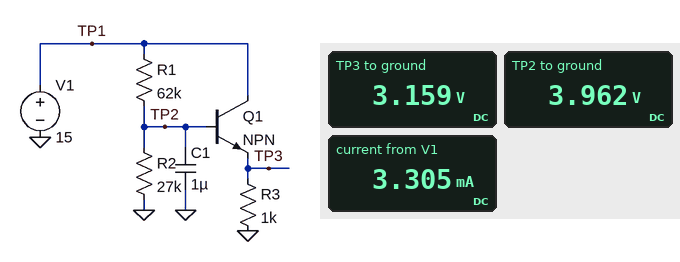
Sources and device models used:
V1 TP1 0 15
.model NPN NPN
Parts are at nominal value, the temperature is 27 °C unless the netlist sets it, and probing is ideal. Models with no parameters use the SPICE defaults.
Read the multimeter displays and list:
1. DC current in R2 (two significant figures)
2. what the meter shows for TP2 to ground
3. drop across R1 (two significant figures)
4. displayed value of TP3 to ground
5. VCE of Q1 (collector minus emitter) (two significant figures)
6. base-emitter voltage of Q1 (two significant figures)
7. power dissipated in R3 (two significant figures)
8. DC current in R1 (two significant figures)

150 µA
3.962 V
11 V
3.159 V
12 V
800 mV
10 mW
180 µA
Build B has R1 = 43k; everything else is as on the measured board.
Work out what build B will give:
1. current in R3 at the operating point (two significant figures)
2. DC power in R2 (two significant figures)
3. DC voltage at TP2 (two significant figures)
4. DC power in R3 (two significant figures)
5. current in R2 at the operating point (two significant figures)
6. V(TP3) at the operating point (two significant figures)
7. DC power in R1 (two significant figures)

4.3 mA
960 µW
5.1 V
18 mW
190 µA
4.3 V
2.3 mW
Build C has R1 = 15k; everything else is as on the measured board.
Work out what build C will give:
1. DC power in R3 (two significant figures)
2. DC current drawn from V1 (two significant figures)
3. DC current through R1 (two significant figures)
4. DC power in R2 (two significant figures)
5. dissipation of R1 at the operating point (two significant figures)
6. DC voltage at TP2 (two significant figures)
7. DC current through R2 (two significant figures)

65 mW
8.4 mA
410 µA
2.9 mW
2.5 mW
8.9 V
330 µA
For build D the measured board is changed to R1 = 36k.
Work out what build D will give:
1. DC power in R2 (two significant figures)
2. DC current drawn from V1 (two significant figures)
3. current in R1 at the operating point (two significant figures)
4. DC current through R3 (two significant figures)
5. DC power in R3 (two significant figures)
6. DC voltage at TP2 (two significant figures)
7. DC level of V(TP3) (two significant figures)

1.2 mW
5.1 mA
260 µA
4.9 mA
24 mW
5.7 V
4.9 V
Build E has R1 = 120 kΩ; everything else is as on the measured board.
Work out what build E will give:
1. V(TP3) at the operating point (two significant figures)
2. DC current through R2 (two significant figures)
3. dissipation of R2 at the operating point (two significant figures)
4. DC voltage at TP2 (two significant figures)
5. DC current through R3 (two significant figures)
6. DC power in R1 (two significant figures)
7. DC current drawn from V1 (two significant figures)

1.6 V
89 µA
210 µW
2.4 V
1.6 mA
1.3 mW
1.7 mA
